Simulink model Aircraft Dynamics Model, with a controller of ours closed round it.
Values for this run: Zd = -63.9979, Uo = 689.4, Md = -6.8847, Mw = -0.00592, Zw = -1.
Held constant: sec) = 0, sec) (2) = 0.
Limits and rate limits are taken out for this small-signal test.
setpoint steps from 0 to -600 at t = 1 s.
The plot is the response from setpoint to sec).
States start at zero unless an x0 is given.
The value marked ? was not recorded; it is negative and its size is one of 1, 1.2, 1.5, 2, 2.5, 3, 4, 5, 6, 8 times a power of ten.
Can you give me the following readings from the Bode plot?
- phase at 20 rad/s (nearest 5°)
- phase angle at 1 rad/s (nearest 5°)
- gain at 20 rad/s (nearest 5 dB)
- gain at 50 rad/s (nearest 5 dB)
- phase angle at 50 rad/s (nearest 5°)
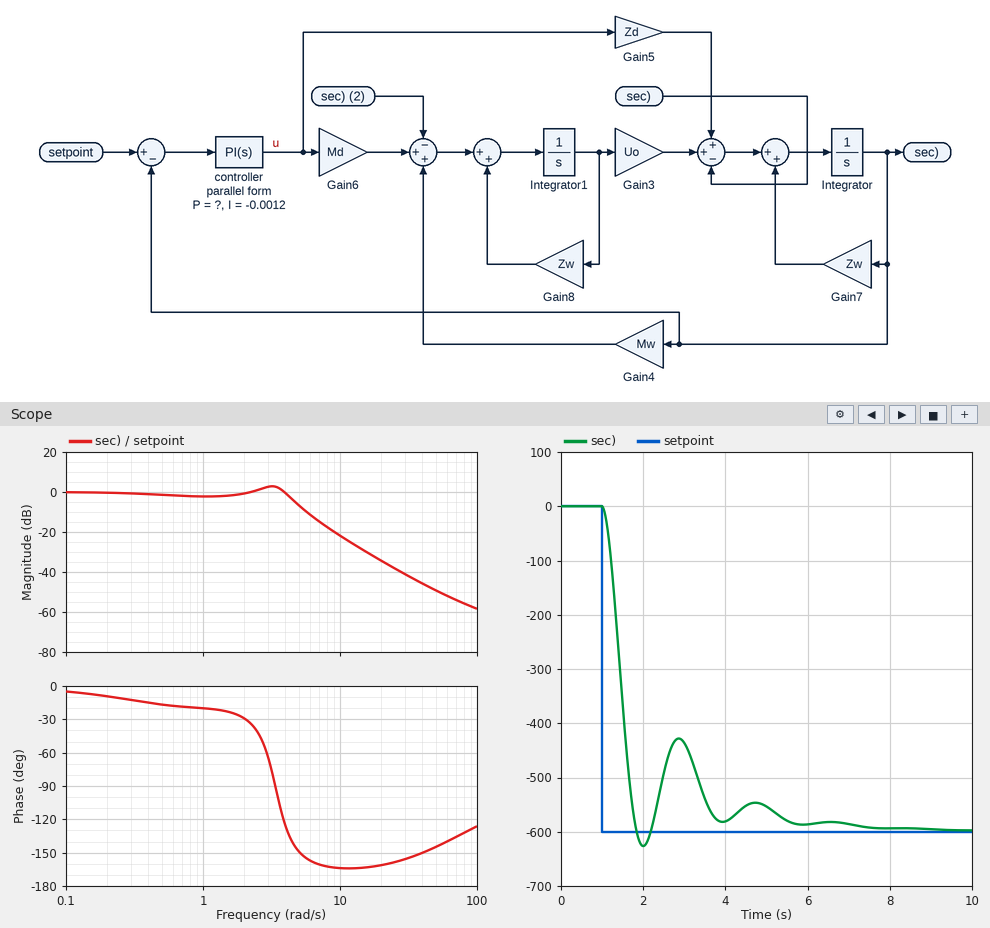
-160°
-20°
-35 dB
-50 dB
-145°
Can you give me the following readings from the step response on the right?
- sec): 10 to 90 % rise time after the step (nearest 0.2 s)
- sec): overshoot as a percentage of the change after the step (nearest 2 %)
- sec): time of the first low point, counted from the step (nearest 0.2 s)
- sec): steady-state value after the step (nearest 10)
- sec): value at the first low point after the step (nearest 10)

0.6 s
4 %
1.0 s
-600
-630
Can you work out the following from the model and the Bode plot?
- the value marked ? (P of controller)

-0.0015
